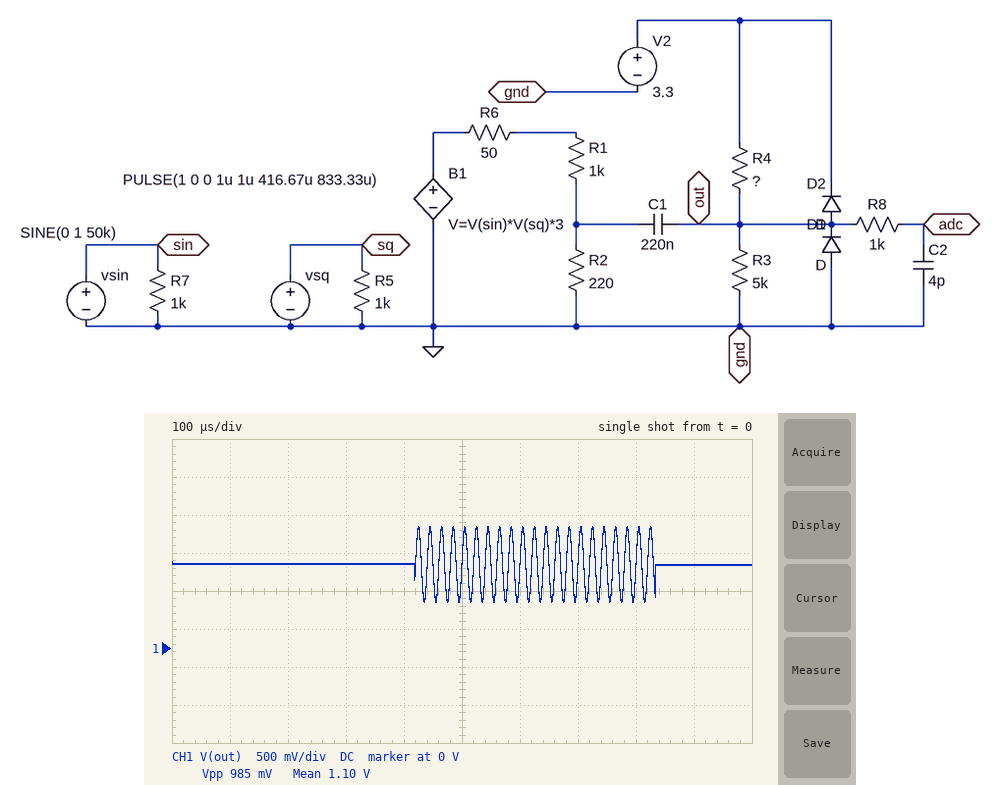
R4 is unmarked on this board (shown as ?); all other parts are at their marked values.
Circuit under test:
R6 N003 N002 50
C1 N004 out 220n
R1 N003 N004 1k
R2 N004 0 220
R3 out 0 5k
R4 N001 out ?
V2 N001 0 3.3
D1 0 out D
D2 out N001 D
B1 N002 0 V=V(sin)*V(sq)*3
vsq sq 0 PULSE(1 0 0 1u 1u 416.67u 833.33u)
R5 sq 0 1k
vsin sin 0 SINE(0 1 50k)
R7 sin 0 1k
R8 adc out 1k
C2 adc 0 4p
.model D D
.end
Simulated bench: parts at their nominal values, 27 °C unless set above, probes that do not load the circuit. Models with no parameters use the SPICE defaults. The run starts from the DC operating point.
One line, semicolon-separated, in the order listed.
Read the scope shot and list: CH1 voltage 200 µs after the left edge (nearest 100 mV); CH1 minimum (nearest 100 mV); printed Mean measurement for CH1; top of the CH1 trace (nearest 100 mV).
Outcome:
1.1 V; 600 mV; 1.10 V; 1.6 V
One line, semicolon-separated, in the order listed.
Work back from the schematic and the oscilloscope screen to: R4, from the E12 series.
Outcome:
10 kΩ
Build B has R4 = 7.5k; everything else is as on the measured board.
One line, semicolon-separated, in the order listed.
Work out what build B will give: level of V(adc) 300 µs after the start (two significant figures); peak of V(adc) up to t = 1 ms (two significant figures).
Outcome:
1.3 V; 1.8 V
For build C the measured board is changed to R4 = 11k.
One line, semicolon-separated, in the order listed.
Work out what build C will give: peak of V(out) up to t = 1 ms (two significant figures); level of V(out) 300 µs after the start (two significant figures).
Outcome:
1.5 V; 1.0 V
